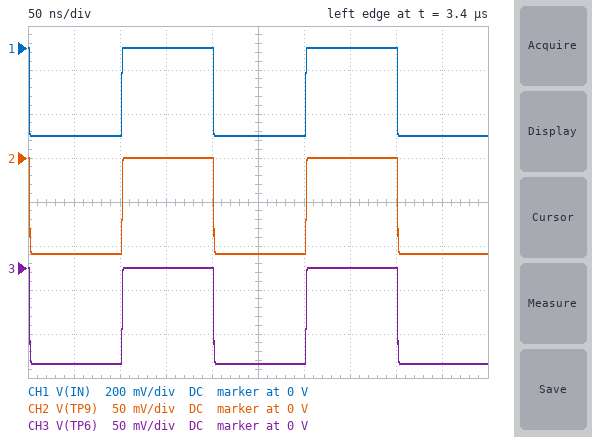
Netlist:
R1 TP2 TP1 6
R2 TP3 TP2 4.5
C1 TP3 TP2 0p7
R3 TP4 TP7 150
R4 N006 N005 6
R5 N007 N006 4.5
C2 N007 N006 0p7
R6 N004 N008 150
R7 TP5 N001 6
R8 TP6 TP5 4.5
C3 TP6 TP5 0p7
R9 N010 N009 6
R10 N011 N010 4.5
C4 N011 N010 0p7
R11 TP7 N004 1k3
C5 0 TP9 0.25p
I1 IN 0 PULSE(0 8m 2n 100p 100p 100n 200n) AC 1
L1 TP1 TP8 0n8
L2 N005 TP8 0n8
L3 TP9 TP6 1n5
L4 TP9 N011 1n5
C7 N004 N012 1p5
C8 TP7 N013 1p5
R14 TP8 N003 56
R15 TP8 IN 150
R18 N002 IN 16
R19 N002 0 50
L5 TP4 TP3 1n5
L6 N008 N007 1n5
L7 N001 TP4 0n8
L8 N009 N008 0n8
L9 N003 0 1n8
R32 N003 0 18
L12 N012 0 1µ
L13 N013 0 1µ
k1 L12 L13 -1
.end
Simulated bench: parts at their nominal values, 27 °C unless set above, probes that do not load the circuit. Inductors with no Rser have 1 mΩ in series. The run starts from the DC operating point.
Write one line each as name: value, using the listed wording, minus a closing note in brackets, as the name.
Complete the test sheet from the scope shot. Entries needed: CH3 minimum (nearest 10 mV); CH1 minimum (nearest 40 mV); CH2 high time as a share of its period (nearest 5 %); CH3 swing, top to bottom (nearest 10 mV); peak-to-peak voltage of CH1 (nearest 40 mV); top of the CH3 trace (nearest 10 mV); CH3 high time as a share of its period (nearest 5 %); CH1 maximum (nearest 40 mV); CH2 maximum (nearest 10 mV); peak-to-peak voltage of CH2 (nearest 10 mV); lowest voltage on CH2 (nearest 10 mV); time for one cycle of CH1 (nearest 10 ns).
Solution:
CH3 minimum: -110 mV
CH1 minimum: -400 mV
CH2 high time as a share of its period: 50 %
CH3 swing, top to bottom: 110 mV
peak-to-peak voltage of CH1: 400 mV
top of the CH3 trace: 0 V
CH3 high time as a share of its period: 50 %
CH1 maximum: 0 V
CH2 maximum: 0 V
peak-to-peak voltage of CH2: 110 mV
lowest voltage on CH2: -110 mV
time for one cycle of CH1: 200 ns
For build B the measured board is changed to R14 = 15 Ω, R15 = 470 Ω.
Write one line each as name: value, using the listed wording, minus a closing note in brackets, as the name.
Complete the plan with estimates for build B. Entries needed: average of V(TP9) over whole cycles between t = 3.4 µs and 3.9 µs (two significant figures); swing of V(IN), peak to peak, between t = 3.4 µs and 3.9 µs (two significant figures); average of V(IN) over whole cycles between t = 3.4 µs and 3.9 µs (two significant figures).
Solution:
average of V(TP9) over whole cycles between t = 3.4 µs and 3.9 µs: -7.2 mV
swing of V(IN), peak to peak, between t = 3.4 µs and 3.9 µs: 470 mV
average of V(IN) over whole cycles between t = 3.4 µs and 3.9 µs: -230 mV
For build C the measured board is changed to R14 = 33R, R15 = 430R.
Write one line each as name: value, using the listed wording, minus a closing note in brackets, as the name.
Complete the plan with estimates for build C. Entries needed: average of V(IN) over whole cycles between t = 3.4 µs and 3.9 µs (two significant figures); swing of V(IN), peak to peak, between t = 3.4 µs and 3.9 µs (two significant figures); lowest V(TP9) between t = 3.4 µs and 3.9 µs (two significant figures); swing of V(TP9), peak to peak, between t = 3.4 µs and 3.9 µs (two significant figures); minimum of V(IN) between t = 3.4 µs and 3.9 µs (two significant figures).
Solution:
average of V(IN) over whole cycles between t = 3.4 µs and 3.9 µs: -230 mV
swing of V(IN), peak to peak, between t = 3.4 µs and 3.9 µs: 460 mV
lowest V(TP9) between t = 3.4 µs and 3.9 µs: -33 mV
swing of V(TP9), peak to peak, between t = 3.4 µs and 3.9 µs: 33 mV
minimum of V(IN) between t = 3.4 µs and 3.9 µs: -460 mV
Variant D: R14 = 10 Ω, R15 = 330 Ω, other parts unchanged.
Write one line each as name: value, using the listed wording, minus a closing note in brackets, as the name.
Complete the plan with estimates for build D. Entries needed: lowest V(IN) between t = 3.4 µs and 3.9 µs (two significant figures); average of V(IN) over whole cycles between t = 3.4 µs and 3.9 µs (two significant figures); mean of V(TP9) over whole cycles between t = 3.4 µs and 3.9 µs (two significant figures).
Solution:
lowest V(IN) between t = 3.4 µs and 3.9 µs: -440 mV
average of V(IN) over whole cycles between t = 3.4 µs and 3.9 µs: -220 mV
mean of V(TP9) over whole cycles between t = 3.4 µs and 3.9 µs: -6.5 mV
